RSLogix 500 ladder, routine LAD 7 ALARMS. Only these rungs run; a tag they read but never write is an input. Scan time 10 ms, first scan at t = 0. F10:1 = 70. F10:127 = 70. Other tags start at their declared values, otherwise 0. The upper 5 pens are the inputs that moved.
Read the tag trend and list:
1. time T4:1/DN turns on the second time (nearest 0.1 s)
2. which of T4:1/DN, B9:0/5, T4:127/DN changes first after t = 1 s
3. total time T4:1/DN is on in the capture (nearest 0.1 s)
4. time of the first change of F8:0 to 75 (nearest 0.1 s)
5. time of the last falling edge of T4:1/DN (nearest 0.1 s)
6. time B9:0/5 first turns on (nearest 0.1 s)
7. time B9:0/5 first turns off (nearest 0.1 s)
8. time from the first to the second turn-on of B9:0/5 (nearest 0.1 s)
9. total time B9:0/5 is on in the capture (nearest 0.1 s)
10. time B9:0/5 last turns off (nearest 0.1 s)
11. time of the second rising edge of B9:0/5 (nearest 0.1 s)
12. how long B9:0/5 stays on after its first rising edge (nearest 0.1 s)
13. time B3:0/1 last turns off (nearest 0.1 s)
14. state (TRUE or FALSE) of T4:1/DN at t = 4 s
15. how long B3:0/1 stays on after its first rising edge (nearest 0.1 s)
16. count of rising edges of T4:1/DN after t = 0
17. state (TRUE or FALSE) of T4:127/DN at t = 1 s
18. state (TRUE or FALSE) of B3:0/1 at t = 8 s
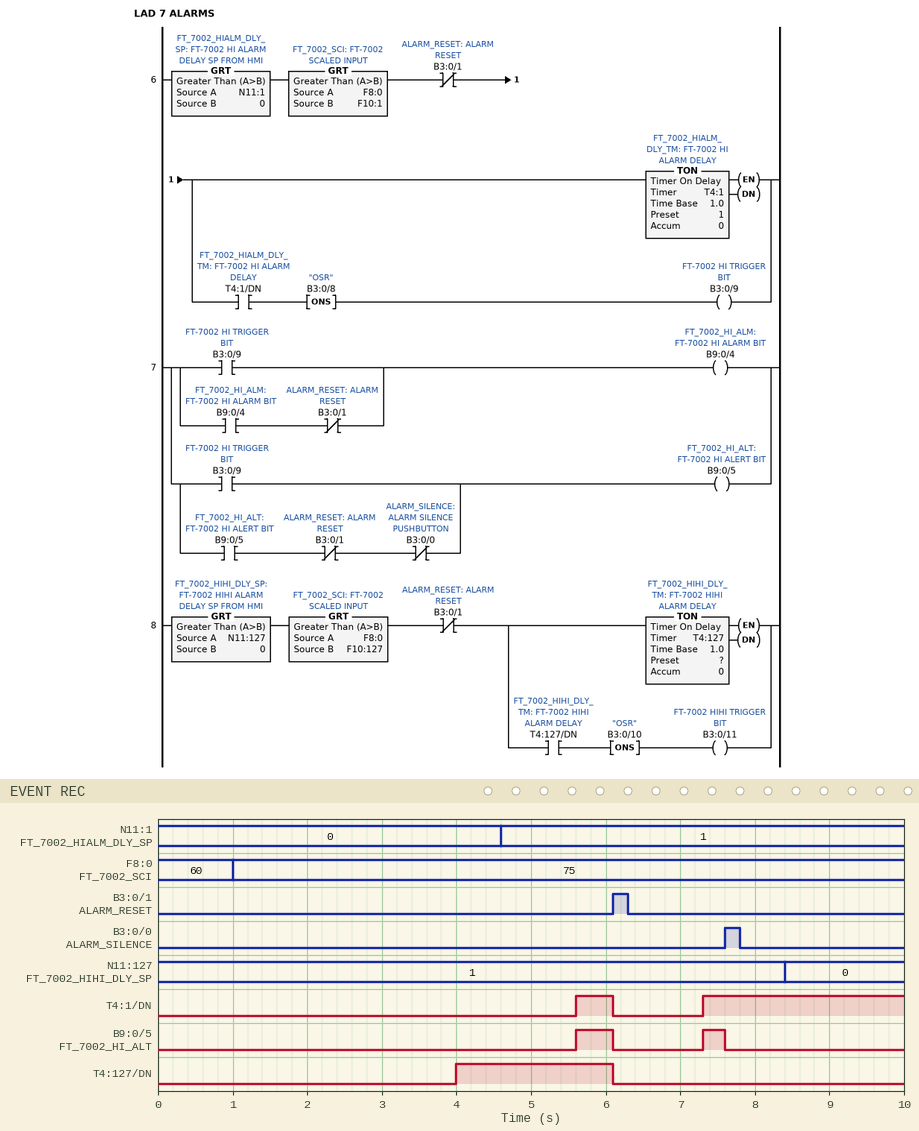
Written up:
7.3 s
T4:127/DN
3.2 s
1.0 s
6.1 s
5.6 s
6.1 s
1.7 s
0.8 s
7.6 s
7.3 s
0.5 s
6.3 s
FALSE
0.2 s
2
FALSE
FALSE
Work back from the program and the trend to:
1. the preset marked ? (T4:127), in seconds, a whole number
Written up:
3 s
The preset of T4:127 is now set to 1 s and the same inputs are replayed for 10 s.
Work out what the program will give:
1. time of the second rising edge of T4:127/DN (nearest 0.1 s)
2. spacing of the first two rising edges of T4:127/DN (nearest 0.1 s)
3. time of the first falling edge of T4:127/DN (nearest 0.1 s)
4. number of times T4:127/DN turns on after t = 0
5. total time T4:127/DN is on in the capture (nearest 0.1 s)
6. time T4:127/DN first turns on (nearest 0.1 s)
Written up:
7.3 s
5.3 s
6.1 s
2
5.2 s
2.0 s
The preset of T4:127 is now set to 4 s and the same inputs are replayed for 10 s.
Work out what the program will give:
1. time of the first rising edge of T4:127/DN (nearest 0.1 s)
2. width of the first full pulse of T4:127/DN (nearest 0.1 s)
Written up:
5.0 s
1.1 s
